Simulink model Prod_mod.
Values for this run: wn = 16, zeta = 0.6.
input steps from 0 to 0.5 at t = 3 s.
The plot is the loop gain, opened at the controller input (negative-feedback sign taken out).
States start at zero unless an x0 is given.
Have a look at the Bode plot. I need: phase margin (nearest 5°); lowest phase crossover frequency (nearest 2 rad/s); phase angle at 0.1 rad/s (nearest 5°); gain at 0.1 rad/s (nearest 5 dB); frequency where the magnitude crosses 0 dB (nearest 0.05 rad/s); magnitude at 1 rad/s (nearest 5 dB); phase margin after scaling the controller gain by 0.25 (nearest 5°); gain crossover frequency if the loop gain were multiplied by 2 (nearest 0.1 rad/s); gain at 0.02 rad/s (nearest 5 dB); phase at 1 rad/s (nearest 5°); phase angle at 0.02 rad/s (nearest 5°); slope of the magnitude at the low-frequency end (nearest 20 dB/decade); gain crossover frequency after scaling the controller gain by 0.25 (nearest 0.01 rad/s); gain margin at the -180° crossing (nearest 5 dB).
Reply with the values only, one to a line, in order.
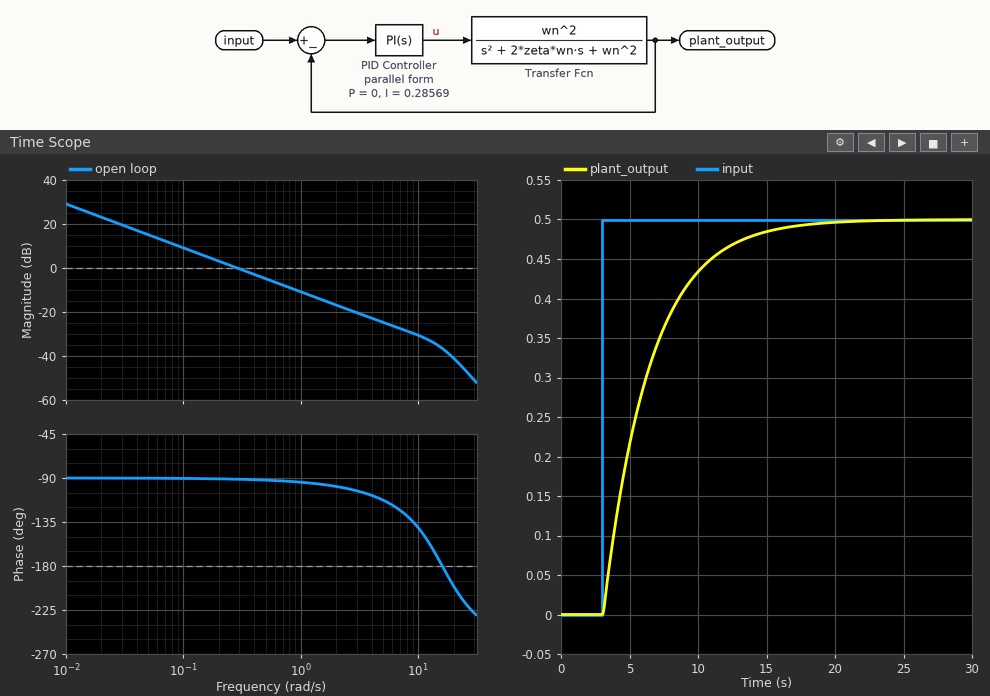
90°
16 rad/s
-90°
10 dB
0.30 rad/s
-10 dB
90°
0.6 rad/s
25 dB
-95°
-90°
-20 dB/decade
0.07 rad/s
35 dB
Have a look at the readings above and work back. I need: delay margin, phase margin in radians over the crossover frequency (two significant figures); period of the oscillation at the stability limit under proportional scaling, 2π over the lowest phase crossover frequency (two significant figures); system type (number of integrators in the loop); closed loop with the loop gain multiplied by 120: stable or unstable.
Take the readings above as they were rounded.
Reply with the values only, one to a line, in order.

5.2 s
0.39 s
1
unstable
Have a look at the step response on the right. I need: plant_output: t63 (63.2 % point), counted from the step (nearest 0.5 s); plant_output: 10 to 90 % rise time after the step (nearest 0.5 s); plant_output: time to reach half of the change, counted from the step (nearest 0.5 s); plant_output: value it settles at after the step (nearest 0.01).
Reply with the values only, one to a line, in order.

3.5 s
7.5 s
2.5 s
0.50
